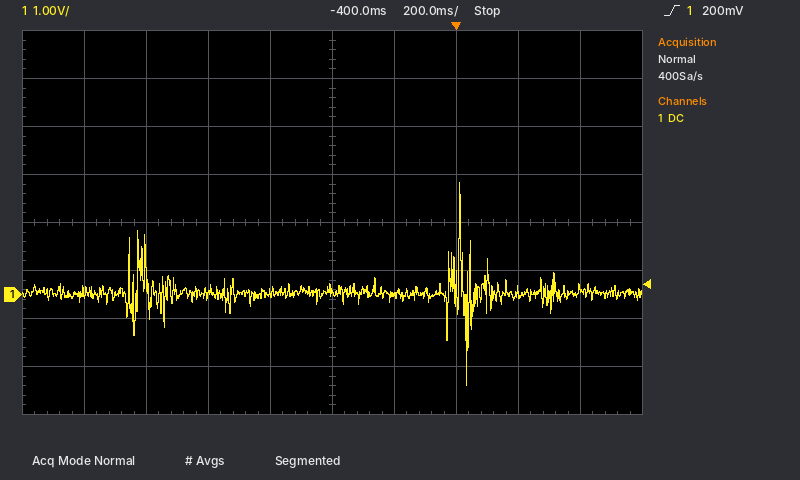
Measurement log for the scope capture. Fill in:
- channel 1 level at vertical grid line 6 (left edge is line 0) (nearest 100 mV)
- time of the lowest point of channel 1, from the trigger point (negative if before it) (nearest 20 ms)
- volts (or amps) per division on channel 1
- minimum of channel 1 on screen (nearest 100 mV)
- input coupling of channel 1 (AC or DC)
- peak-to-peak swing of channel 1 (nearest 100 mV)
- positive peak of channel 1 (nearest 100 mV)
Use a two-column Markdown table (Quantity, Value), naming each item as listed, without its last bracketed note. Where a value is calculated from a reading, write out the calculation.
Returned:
| Quantity | Value |
|---|---|
| channel 1 level at vertical grid line 6 (left edge is line 0) | 0.0 V |
| time of the lowest point of channel 1, from the trigger point (negative if before it) | +40 ms |
| volts (or amps) per division on channel 1 | 1 V |
| minimum of channel 1 on screen | -1.9 V |
| input coupling of channel 1 | DC |
| peak-to-peak swing of channel 1 | 2.3 V − (-1.9 V) = 4.2 V |
| positive peak of channel 1 | 2.3 V |
